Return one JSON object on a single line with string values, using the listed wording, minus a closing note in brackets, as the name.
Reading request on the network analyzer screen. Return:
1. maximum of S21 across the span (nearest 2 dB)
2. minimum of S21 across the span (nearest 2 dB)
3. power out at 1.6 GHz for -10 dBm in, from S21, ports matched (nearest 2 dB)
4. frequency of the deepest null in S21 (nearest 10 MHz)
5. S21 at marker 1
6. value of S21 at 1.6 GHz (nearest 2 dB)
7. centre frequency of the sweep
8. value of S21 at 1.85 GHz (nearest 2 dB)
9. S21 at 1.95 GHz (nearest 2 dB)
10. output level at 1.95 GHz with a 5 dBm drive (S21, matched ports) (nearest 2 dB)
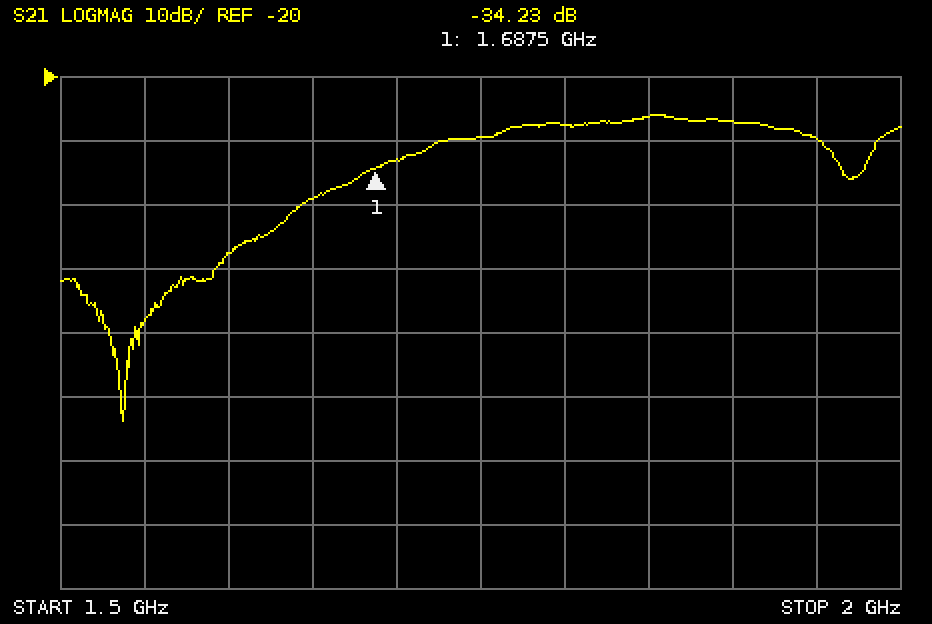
{"maximum of S21 across the span": "-26 dB", "minimum of S21 across the span": "-74 dB", "power out at 1.6 GHz for -10 dBm in, from S21, ports matched": "-58 dBm", "frequency of the deepest null in S21": "1.54 GHz", "S21 at marker 1": "-34.23 dB", "value of S21 at 1.6 GHz": "-48 dB", "centre frequency of the sweep": "1.75 GHz", "value of S21 at 1.85 GHz": "-26 dB", "S21 at 1.95 GHz": "-30 dB", "output level at 1.95 GHz with a 5 dBm drive (S21, matched ports)": "-24 dBm"}
